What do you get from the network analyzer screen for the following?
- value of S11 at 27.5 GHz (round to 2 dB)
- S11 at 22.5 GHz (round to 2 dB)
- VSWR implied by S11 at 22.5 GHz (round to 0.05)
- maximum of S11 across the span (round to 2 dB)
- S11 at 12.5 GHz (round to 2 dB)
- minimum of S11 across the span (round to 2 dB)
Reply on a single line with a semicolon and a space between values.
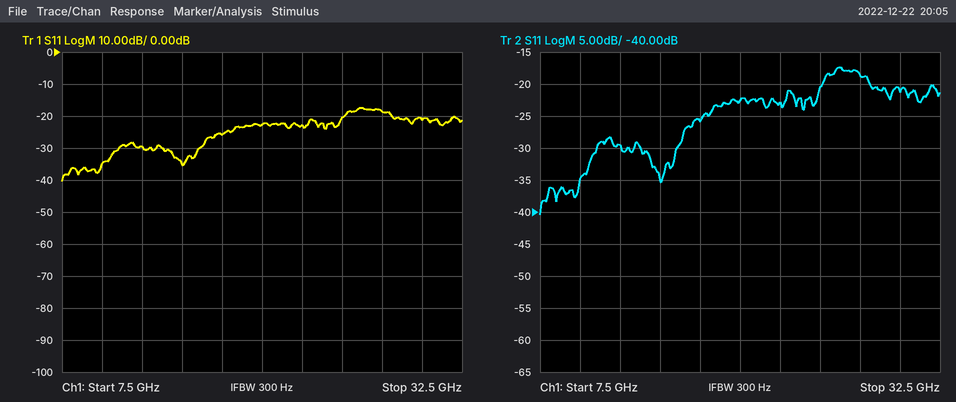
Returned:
-18 dB; -22 dB; 1.15; -18 dB; -30 dB; -40 dB
